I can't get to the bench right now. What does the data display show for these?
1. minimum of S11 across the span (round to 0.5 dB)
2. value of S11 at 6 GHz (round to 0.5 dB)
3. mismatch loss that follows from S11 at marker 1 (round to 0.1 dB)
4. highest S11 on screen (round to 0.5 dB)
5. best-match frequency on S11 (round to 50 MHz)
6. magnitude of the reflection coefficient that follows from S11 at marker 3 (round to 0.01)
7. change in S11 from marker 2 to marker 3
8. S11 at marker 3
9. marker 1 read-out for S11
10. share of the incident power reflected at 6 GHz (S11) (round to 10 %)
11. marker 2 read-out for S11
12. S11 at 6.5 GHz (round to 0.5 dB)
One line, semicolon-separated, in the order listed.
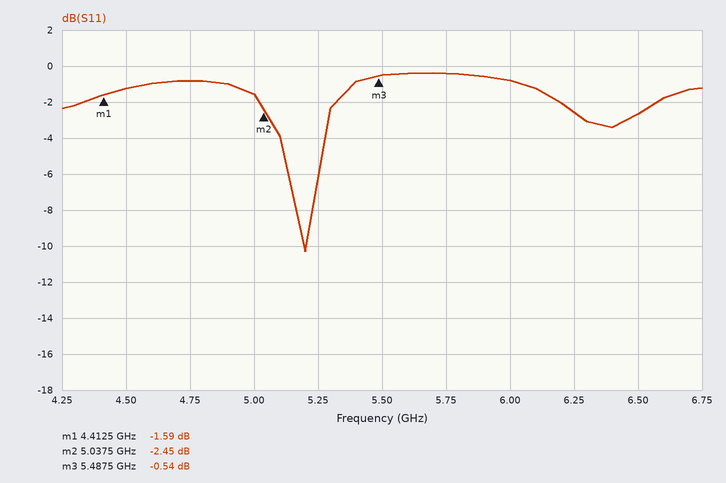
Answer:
-10.5 dB; -1.0 dB; 5.1 dB; -0.5 dB; 5.20 GHz; 0.94; 1.91 dB; -0.54 dB; -1.59 dB; 80 %; -2.45 dB; -2.5 dB
